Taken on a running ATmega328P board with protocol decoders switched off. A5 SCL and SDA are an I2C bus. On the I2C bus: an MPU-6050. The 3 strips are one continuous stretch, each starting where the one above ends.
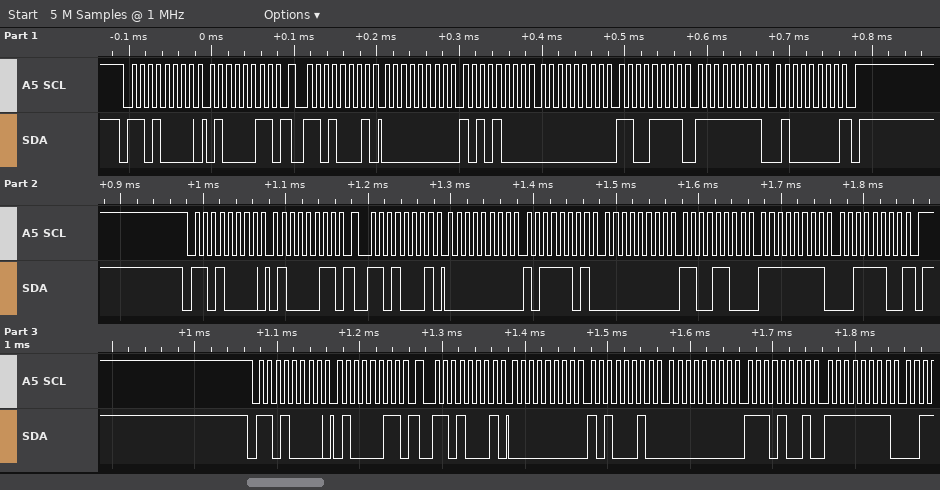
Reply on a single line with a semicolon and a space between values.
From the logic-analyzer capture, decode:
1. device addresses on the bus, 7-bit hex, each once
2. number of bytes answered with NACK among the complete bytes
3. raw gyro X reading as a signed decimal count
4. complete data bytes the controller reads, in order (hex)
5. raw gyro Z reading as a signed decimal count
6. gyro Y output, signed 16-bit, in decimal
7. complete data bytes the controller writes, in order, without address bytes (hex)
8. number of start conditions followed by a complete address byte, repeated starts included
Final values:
0x68; 2; 168; 00 A8 00 CF FF 40 00 BD 00 CC FF 3C 00 A2 00 E9 FF; -192; 207; 43 43 43; 6
